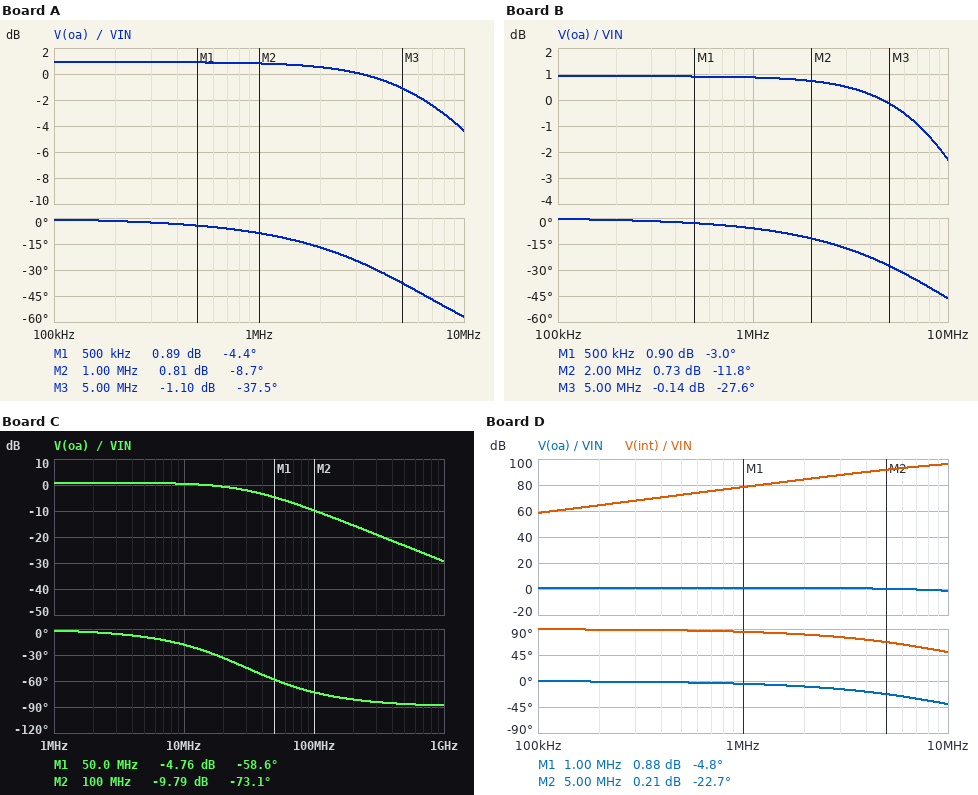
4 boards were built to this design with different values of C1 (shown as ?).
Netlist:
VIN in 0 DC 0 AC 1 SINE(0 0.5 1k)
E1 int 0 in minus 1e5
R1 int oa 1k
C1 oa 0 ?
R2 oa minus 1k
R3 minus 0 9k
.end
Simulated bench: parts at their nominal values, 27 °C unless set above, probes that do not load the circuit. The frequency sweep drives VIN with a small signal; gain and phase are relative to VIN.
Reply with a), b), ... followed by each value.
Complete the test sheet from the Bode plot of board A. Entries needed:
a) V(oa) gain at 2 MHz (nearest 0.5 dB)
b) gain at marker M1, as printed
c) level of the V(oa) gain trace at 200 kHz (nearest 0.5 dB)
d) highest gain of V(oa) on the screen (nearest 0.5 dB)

a) 0.5 dB
b) 0.89 dB
c) 1.0 dB
d) 1.0 dB
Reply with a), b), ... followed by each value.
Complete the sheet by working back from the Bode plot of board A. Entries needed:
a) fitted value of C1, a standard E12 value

a) 2.2 µF
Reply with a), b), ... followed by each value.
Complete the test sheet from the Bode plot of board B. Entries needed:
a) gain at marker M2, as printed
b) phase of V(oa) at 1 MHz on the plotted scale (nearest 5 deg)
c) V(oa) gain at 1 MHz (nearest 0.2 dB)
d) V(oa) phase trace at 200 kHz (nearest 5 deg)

a) 0.73 dB
b) -5 deg
c) 0.8 dB
d) 0 deg
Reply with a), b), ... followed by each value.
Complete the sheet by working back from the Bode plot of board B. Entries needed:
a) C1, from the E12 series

a) 1.5 µF
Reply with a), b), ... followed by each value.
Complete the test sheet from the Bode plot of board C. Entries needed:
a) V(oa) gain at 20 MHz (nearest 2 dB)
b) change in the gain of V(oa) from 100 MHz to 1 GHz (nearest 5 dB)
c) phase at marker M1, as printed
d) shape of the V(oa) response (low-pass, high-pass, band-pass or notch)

a) 0 dB
b) -20 dB
c) -58.6 deg
d) low-pass
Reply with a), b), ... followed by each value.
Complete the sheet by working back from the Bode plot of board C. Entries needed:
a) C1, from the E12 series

a) 470 nF
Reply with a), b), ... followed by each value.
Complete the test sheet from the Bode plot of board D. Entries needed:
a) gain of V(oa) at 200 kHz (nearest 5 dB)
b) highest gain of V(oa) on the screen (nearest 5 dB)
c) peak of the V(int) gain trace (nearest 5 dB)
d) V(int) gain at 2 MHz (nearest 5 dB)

a) 0 dB
b) 0 dB
c) 95 dB
d) 85 dB
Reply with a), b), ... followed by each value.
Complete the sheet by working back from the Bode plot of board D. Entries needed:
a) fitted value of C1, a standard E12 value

a) 1.2 µF
